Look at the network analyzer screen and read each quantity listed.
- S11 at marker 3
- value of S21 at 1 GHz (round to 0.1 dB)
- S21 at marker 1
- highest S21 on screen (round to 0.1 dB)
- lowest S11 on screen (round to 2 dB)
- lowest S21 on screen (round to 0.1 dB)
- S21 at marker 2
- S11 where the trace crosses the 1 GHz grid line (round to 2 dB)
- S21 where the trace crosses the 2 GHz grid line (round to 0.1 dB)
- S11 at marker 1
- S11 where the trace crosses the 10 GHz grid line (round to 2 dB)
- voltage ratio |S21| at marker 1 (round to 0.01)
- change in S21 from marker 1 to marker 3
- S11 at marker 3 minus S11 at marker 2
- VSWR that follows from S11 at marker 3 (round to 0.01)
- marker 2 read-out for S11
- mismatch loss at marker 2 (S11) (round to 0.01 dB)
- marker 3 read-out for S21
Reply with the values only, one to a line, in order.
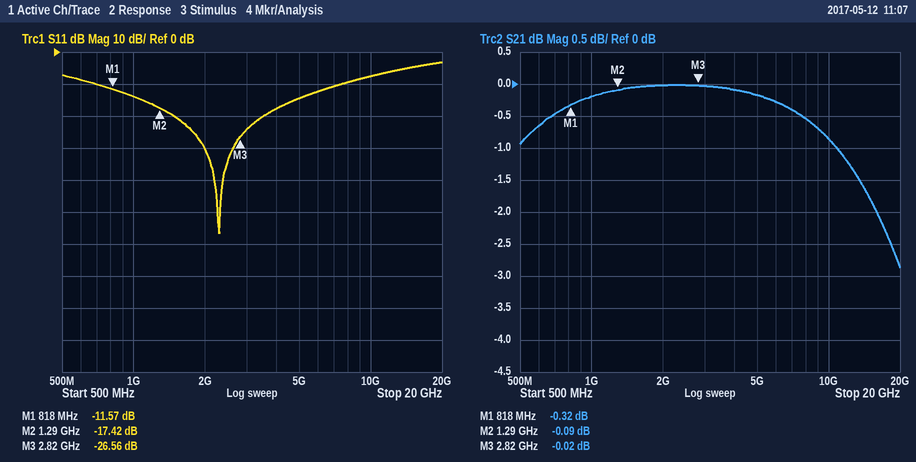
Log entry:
-26.56 dB
-0.2 dB
-0.32 dB
0.0 dB
-56 dB
-2.9 dB
-0.09 dB
-14 dB
0.0 dB
-11.57 dB
-8 dB
0.96
0.30 dB
-9.14 dB
1.10
-17.42 dB
0.08 dB
-0.02 dB
